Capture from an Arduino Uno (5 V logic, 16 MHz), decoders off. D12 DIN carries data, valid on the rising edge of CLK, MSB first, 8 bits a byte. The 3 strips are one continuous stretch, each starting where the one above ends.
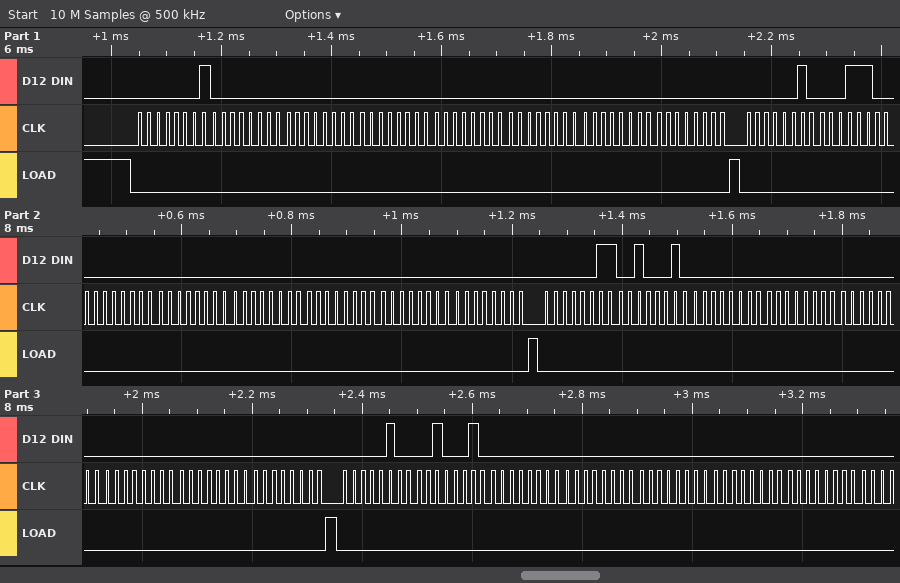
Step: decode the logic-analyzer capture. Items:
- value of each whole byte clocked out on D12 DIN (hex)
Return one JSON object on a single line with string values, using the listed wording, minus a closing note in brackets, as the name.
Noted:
{"value of each whole byte clocked out on D12 DIN": "01 00 00 00 00 00 00 00 02 1C 00 00 00 00 00 00 03 22 00 00 00 00 00 00 04 22 00 00 00 00 00"}
